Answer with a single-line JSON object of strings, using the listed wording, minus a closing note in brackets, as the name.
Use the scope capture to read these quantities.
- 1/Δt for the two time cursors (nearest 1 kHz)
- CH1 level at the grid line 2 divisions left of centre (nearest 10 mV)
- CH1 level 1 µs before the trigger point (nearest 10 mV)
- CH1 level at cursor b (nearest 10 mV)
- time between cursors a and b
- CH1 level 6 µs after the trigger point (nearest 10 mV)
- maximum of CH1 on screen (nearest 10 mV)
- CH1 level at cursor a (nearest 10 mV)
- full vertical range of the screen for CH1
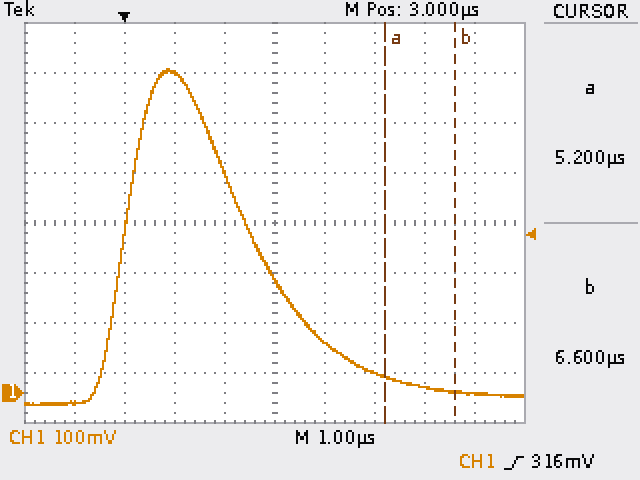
{"1/Δt for the two time cursors": "714 kHz", "CH1 level at the grid line 2 divisions left of centre": "640 mV", "CH1 level 1 µs before the trigger point": "-20 mV", "CH1 level at cursor b": "0 mV", "time between cursors a and b": "1.4 µs", "CH1 level 6 µs after the trigger point": "10 mV", "maximum of CH1 on screen": "650 mV", "CH1 level at cursor a": "30 mV", "full vertical range of the screen for CH1": "800 mV"}
